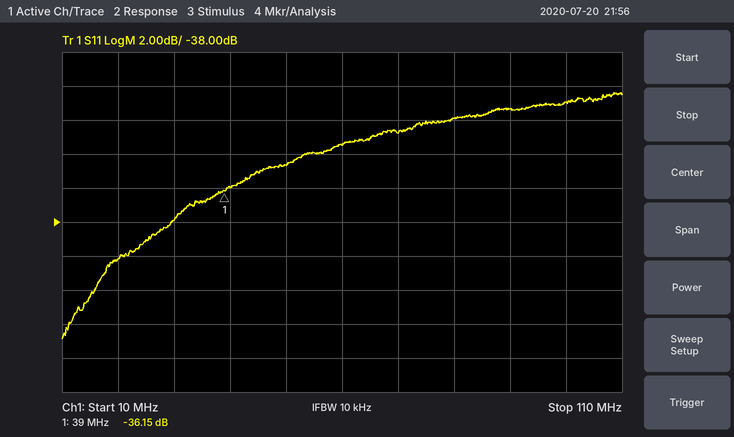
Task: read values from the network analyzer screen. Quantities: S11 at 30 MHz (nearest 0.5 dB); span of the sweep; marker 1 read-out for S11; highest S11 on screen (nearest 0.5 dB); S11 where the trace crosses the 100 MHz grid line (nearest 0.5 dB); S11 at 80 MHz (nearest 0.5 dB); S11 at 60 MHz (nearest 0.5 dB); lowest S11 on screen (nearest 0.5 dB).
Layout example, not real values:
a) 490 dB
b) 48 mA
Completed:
a) -38.0 dB
b) 100 MHz
c) -36.15 dB
d) -30.5 dB
e) -31.0 dB
f) -32.0 dB
g) -33.5 dB
h) -45.0 dB
